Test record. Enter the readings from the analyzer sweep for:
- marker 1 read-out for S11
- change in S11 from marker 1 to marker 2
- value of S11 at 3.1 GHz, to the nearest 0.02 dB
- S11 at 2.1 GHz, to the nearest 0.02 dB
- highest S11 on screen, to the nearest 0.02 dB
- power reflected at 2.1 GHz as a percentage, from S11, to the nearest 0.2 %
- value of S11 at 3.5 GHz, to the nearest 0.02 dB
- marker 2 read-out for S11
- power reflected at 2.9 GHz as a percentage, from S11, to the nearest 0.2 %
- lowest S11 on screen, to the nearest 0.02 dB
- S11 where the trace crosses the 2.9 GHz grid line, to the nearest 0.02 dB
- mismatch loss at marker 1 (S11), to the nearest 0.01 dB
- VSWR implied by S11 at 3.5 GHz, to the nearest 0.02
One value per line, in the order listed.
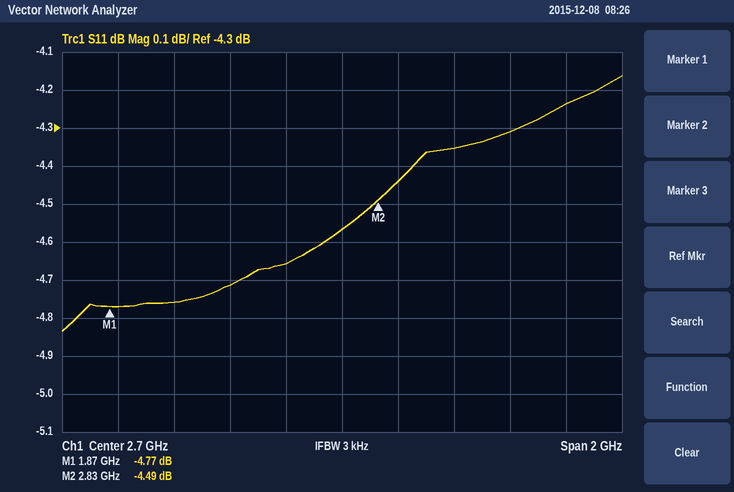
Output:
-4.77 dB
0.28 dB
-4.36 dB
-4.76 dB
-4.16 dB
33.4 %
-4.24 dB
-4.49 dB
36.0 %
-4.84 dB
-4.44 dB
1.76 dB
4.18
